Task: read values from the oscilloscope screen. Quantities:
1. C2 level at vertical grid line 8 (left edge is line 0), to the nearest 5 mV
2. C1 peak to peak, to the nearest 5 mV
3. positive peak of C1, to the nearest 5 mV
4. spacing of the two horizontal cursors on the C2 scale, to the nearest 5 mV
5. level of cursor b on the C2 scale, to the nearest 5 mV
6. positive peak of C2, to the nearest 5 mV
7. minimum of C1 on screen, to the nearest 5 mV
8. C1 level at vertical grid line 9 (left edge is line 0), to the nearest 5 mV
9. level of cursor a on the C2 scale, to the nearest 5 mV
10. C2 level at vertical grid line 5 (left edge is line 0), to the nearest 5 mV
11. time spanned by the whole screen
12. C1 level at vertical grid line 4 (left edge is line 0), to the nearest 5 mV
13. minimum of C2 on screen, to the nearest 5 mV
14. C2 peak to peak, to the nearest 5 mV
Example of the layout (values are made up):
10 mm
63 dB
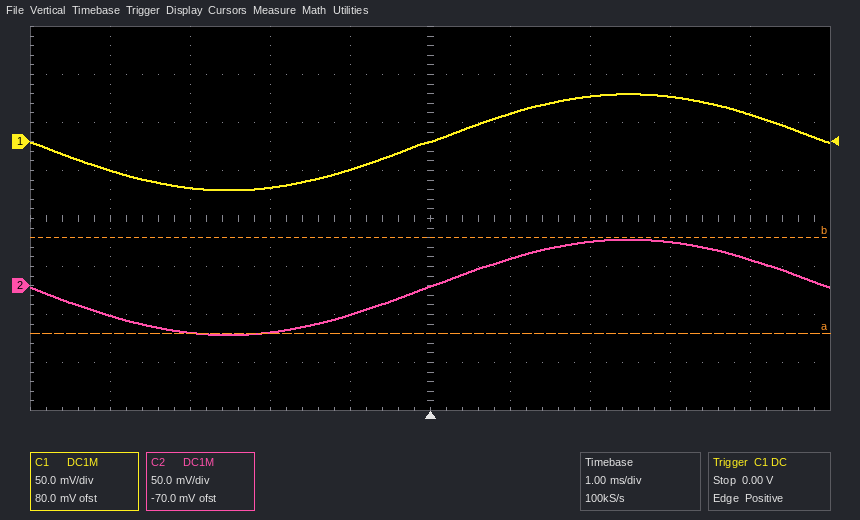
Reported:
45 mV
100 mV
50 mV
100 mV
50 mV
50 mV
-50 mV
30 mV
-50 mV
0 mV
10 ms
-30 mV
-50 mV
100 mV
